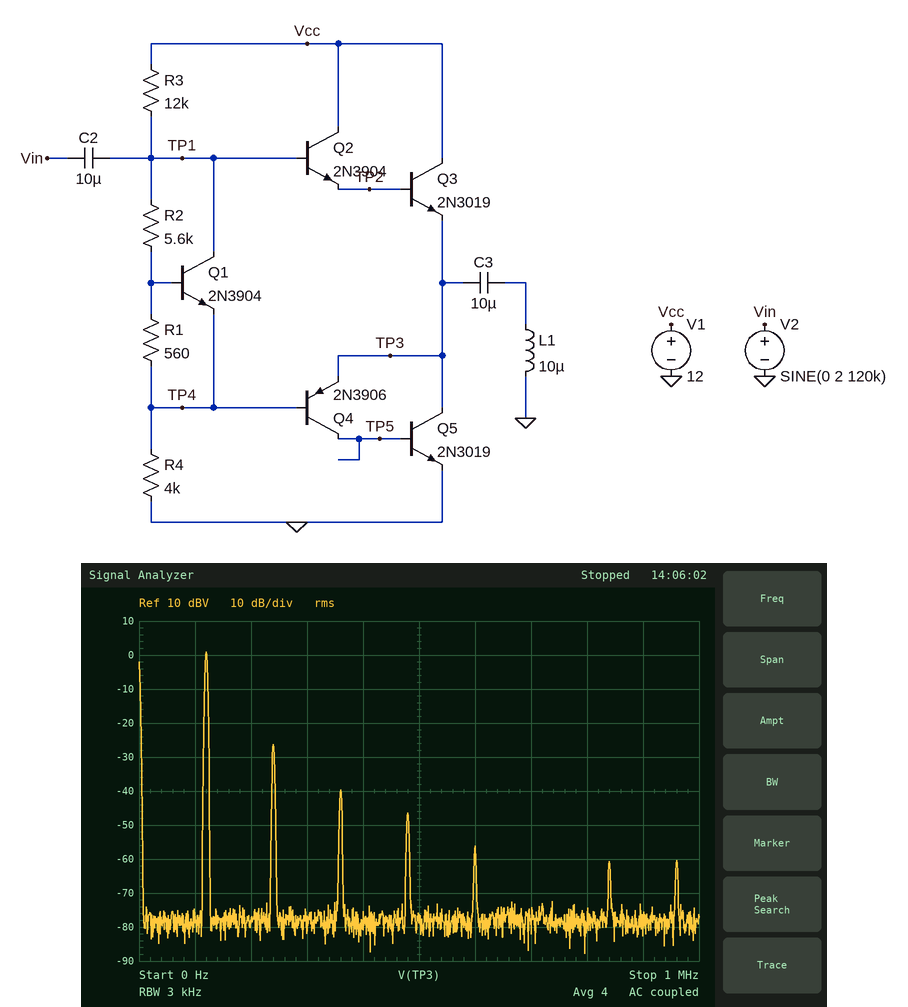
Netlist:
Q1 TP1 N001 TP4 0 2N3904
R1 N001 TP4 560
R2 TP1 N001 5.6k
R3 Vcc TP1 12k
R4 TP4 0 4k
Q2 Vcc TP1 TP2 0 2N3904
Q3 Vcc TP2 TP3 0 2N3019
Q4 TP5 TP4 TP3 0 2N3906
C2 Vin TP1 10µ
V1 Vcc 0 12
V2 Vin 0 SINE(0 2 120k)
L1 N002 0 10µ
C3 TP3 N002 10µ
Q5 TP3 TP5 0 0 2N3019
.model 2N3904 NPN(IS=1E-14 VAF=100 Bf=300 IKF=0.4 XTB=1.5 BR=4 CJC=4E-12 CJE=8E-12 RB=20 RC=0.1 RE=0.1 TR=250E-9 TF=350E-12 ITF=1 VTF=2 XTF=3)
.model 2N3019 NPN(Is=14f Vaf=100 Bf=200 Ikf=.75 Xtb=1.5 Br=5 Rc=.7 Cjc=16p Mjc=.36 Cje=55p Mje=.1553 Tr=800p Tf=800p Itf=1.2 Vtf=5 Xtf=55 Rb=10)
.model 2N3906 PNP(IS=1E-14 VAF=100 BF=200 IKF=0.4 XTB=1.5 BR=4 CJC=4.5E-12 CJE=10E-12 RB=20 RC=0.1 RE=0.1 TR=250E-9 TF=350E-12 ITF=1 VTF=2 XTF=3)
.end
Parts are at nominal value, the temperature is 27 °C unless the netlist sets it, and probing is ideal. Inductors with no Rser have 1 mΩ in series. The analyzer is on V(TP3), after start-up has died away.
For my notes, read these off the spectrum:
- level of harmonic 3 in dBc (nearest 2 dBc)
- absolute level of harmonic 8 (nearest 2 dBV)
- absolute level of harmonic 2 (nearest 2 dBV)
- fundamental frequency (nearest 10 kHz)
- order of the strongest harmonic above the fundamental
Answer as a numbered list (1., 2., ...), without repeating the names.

1. -40 dBc
2. -60 dBV
3. -26 dBV
4. 120 kHz
5. 2
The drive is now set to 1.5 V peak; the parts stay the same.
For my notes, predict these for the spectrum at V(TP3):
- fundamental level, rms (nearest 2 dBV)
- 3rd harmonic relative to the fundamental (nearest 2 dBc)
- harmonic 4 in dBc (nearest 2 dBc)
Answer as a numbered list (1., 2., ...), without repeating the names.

1. -2 dBV
2. -52 dBc
3. -58 dBc
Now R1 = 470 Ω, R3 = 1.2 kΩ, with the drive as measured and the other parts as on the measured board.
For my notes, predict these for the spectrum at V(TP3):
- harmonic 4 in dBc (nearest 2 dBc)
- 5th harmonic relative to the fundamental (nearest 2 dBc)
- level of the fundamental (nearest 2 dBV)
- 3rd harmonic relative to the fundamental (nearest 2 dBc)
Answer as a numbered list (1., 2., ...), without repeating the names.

1. -42 dBc
2. -44 dBc
3. 0 dBV
4. -38 dBc
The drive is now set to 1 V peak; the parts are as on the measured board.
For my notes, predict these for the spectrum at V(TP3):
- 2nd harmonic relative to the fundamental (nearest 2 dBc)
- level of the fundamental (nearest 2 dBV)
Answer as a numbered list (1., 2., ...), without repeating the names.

1. -36 dBc
2. -6 dBV
